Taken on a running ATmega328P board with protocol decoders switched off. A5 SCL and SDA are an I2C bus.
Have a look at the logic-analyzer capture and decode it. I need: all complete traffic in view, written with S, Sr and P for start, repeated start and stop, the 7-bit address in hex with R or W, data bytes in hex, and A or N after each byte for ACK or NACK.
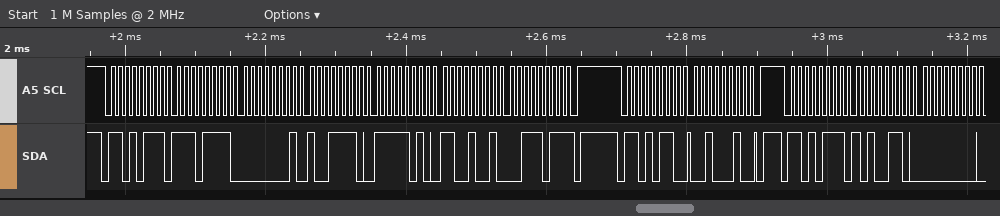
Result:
S 6BR A EF A 01 A 9E A FA A C9 A 3B N P S 6BW A 22 A P S 6BR A A6 A 00 A
